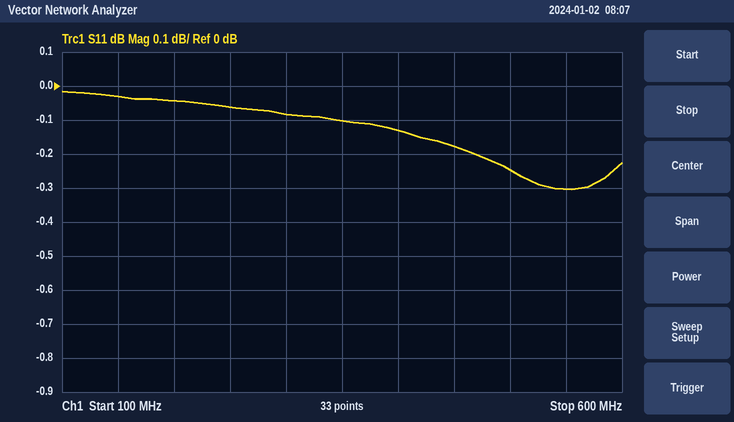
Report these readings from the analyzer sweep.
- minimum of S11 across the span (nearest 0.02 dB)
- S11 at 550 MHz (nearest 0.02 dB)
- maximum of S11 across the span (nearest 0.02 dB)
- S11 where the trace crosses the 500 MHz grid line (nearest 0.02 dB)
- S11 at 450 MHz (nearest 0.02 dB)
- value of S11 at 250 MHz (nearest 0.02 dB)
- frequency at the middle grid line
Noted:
-0.30 dB
-0.30 dB
-0.02 dB
-0.24 dB
-0.18 dB
-0.06 dB
350 MHz
